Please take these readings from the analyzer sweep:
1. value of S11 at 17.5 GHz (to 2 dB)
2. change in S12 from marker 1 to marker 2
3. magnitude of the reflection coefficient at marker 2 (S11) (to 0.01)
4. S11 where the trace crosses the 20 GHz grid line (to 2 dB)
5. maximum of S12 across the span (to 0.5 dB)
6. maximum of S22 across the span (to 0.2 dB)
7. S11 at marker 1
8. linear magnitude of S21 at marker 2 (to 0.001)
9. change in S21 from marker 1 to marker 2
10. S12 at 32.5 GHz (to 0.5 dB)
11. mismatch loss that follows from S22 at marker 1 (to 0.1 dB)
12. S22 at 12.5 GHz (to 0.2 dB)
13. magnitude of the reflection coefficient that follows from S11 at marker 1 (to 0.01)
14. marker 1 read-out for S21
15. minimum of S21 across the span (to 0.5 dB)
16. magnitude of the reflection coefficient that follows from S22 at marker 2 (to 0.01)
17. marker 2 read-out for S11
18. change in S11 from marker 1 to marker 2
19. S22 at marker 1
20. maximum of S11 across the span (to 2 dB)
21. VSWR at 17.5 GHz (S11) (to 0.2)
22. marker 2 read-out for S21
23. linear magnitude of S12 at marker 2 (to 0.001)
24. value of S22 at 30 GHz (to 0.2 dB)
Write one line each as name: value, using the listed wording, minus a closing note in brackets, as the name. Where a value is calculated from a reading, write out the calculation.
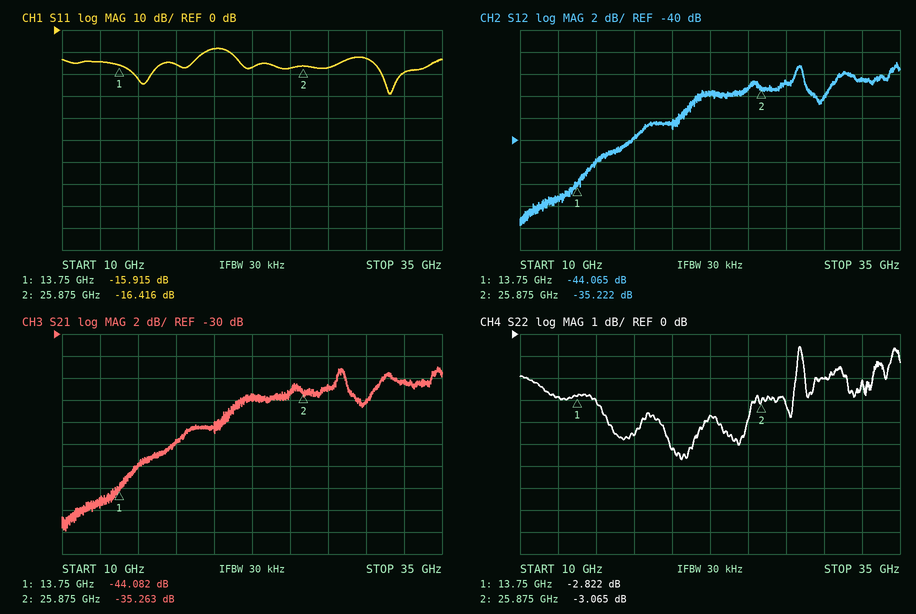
value of S11 at 17.5 GHz: -16 dB
change in S12 from marker 1 to marker 2: -35.222 − (-44.065) = 8.843 dB
magnitude of the reflection coefficient at marker 2 (S11): 10^(-16.416/20) ≈ 0.15
S11 where the trace crosses the 20 GHz grid line: -8 dB
maximum of S12 across the span: -33.0 dB
maximum of S22 across the span: -0.6 dB
S11 at marker 1: -15.915 dB
linear magnitude of S21 at marker 2: 10^(-35.263/20) ≈ 0.017
change in S21 from marker 1 to marker 2: -35.263 − (-44.082) = 8.819 dB
S12 at 32.5 GHz: -34.5 dB
mismatch loss that follows from S22 at marker 1: −10 log10(1 − 10^(-2.822/10)) ≈ 3.2 dB
S22 at 12.5 GHz: -2.8 dB
magnitude of the reflection coefficient that follows from S11 at marker 1: 10^(-15.915/20) ≈ 0.16
marker 1 read-out for S21: -44.082 dB
minimum of S21 across the span: -48.0 dB
magnitude of the reflection coefficient that follows from S22 at marker 2: 10^(-3.065/20) ≈ 0.70
marker 2 read-out for S11: -16.416 dB
change in S11 from marker 1 to marker 2: -16.416 − (-15.915) = -0.501 dB
S22 at marker 1: -2.822 dB
maximum of S11 across the span: -8 dB
VSWR at 17.5 GHz (S11): |Γ| = 10^(-16/20) = 0.1585; VSWR = (1 + 0.1585)/(1 − 0.1585) ≈ 1.4
marker 2 read-out for S21: -35.263 dB
linear magnitude of S12 at marker 2: 10^(-35.222/20) ≈ 0.017
value of S22 at 30 GHz: -2.0 dB
